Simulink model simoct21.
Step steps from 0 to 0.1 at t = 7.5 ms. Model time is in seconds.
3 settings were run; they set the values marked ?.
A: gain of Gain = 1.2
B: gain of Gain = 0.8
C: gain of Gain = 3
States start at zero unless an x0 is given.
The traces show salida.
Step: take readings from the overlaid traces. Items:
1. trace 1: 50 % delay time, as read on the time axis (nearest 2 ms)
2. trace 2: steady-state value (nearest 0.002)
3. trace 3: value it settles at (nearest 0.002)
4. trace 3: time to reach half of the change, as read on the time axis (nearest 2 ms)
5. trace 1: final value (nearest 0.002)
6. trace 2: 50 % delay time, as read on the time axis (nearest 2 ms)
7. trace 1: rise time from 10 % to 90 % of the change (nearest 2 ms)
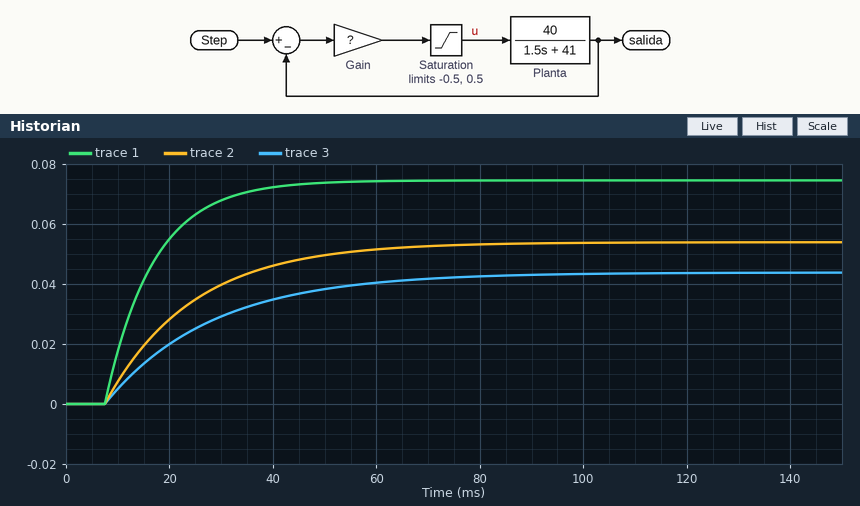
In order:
14 ms
0.054
0.044
22 ms
0.074
20 ms
20 ms
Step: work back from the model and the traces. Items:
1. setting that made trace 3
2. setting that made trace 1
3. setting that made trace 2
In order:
B
C
A
